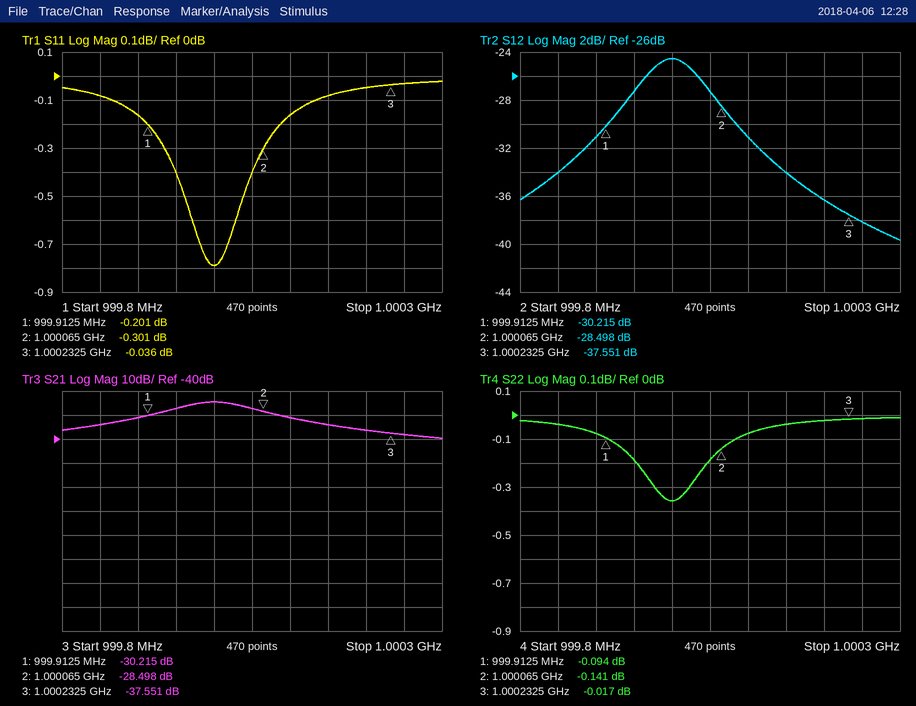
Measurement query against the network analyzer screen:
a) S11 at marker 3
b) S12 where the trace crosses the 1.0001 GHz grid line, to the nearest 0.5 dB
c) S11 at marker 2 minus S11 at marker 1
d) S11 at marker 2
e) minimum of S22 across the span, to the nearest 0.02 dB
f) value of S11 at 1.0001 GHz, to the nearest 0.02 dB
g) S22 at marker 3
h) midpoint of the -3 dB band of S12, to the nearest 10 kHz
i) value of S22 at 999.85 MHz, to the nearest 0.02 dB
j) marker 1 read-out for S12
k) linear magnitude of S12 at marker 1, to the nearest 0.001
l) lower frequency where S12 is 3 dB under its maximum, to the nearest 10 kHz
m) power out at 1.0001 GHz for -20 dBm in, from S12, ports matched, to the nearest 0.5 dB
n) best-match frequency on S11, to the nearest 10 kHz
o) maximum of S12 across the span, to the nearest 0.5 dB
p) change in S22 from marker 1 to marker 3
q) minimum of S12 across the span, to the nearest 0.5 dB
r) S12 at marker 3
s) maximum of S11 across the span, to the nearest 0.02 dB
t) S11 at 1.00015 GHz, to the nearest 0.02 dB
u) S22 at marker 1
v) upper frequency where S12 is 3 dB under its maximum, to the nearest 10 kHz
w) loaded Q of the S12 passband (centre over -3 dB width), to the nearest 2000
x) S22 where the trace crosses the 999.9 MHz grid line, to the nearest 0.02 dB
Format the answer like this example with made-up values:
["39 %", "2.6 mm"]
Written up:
["-0.036 dB", "-31.0 dB", "-0.100 dB", "-0.301 dB", "-0.36 dB", "-0.16 dB", "-0.017 dB", "1.00000 GHz", "-0.04 dB", "-30.215 dB", "0.031", "999.95 MHz", "-51.0 dBm", "1.00000 GHz", "-24.5 dB", "0.077 dB", "-39.5 dB", "-37.551 dB", "-0.02 dB", "-0.08 dB", "-0.094 dB", "1.00005 GHz", "10000", "-0.08 dB"]
